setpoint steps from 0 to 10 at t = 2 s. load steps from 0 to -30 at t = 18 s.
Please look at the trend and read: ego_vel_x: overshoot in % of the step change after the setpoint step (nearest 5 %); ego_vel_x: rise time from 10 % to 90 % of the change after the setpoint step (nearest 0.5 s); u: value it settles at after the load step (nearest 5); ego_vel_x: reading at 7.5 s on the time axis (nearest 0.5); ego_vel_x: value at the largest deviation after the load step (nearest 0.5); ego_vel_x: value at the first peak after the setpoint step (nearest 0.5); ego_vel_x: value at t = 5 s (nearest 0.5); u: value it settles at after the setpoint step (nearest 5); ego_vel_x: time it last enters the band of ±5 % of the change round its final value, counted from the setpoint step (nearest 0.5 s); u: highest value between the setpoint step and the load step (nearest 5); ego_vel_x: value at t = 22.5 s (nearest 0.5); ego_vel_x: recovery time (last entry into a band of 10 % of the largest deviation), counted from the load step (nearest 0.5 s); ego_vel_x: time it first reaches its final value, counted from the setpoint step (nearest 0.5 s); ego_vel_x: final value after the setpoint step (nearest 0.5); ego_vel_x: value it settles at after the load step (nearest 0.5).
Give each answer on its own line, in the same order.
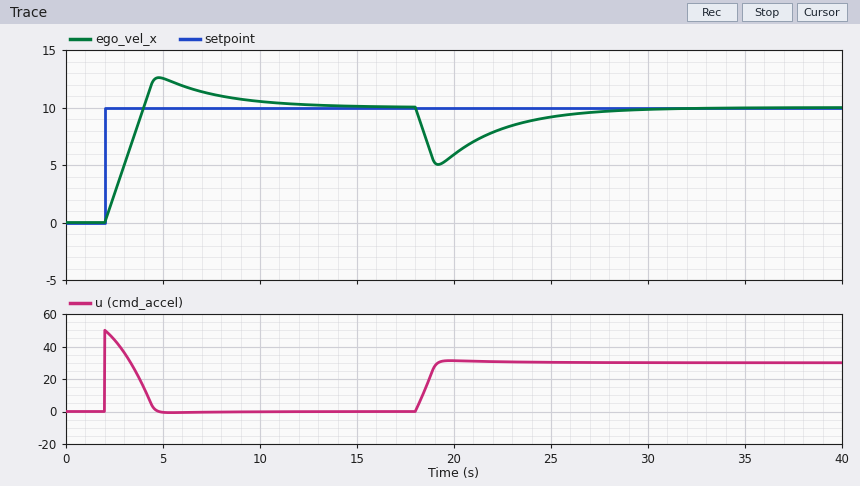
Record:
25 %
1.5 s
30
11.0
5.0
12.5
12.5
0
8.0 s
50
8.0
8.5 s
2.0 s
10.0
10.0
